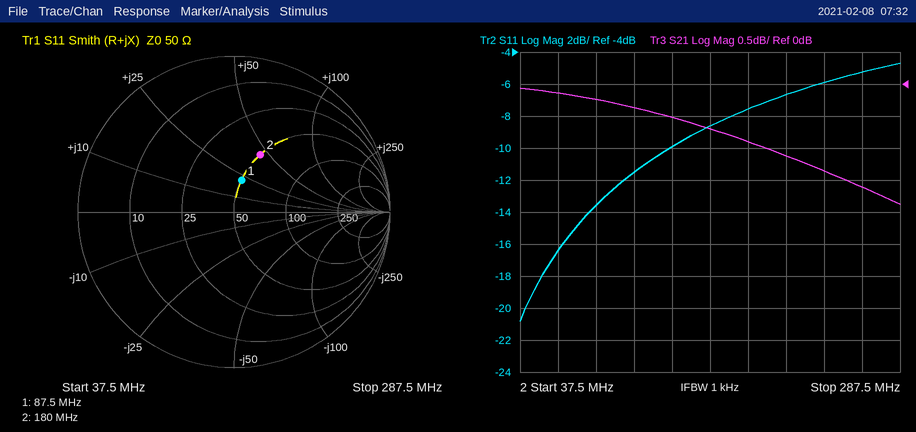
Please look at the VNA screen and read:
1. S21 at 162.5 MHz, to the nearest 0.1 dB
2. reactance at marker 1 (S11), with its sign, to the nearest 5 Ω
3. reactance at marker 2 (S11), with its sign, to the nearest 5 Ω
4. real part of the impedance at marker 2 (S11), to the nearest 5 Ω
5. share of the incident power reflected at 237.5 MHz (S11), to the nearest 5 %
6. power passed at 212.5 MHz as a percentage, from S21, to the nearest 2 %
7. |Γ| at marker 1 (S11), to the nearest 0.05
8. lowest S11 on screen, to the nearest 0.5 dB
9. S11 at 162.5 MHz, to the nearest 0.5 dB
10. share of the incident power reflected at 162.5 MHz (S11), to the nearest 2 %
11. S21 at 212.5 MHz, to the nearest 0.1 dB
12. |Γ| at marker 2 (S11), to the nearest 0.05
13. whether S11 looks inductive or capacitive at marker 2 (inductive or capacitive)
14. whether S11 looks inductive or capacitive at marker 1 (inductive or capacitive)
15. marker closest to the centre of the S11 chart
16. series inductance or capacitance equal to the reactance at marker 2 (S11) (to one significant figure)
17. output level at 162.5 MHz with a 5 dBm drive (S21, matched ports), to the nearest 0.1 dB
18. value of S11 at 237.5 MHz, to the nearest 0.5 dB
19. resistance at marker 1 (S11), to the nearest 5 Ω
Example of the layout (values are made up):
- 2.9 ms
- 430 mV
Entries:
- -0.7 dB
- +20 Ω
- +45 Ω
- 50 Ω
- 25 %
- 78 %
- 0.20
- -21.0 dB
- -8.5 dB
- 14 %
- -1.1 dB
- 0.40
- inductive
- inductive
- marker 1
- 40 nH
- 4.3 dBm
- -6.0 dB
- 50 Ω
